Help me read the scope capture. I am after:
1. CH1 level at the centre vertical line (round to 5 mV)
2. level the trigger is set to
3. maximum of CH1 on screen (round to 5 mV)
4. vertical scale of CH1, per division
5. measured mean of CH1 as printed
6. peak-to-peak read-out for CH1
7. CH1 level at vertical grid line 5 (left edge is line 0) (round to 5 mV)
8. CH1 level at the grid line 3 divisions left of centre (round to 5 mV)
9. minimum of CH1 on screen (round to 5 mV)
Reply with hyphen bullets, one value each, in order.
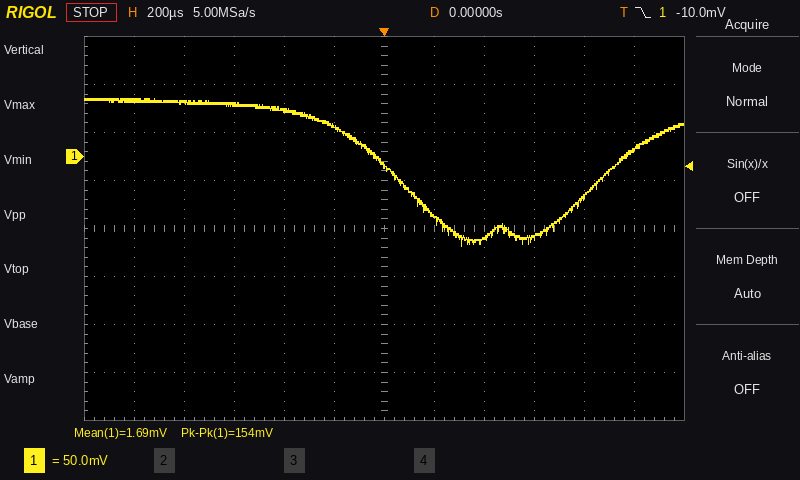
- -10 mV
- -10.0 mV
- 60 mV
- 50 mV
- 1.69 mV
- 154 mV
- 30 mV
- 55 mV
- -95 mV
